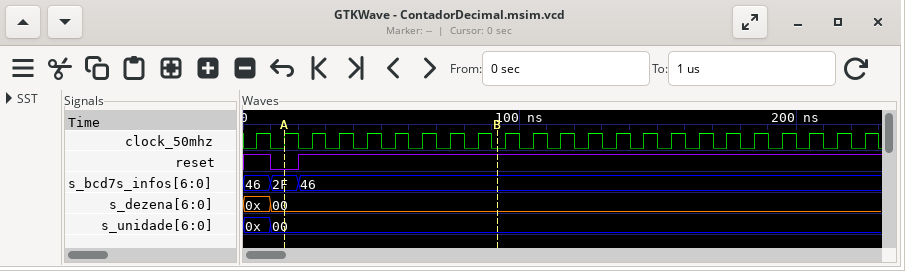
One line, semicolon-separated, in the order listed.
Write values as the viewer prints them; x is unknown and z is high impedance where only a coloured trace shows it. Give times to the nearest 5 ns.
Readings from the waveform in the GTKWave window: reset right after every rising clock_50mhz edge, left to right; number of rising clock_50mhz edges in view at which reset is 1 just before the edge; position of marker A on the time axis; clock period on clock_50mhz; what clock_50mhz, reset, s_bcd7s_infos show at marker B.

1 0 1 1 1 1 1 1 1 1 1 1 1 1 1 1 1 1 1 1 1 1 1; 22; 15 ns; 10 ns; clock_50mhz=0, reset=1, s_bcd7s_infos=46
